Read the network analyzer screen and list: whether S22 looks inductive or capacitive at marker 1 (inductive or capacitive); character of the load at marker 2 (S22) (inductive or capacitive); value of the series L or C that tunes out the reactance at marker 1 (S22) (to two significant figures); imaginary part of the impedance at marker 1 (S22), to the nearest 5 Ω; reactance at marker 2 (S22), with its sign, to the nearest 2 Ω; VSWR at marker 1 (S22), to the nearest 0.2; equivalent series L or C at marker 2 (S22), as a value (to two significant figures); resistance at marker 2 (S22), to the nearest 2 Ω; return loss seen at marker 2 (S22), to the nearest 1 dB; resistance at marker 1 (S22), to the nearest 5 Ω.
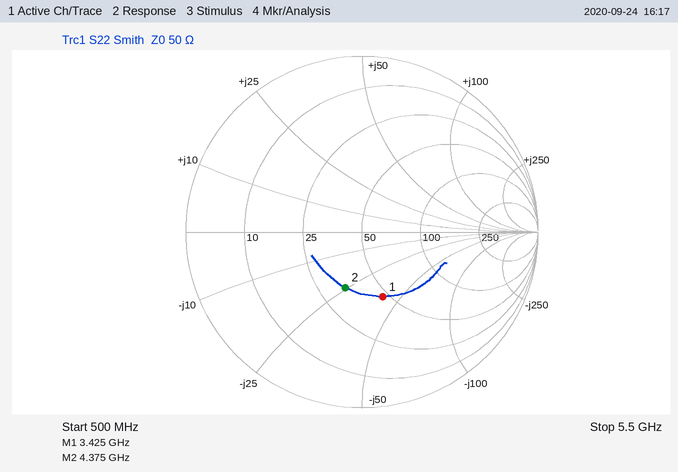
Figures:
capacitive
capacitive
1.9 nH
-40 Ω
-24 Ω
2.2
1.5 pF
34 Ω
10 dB
45 Ω
